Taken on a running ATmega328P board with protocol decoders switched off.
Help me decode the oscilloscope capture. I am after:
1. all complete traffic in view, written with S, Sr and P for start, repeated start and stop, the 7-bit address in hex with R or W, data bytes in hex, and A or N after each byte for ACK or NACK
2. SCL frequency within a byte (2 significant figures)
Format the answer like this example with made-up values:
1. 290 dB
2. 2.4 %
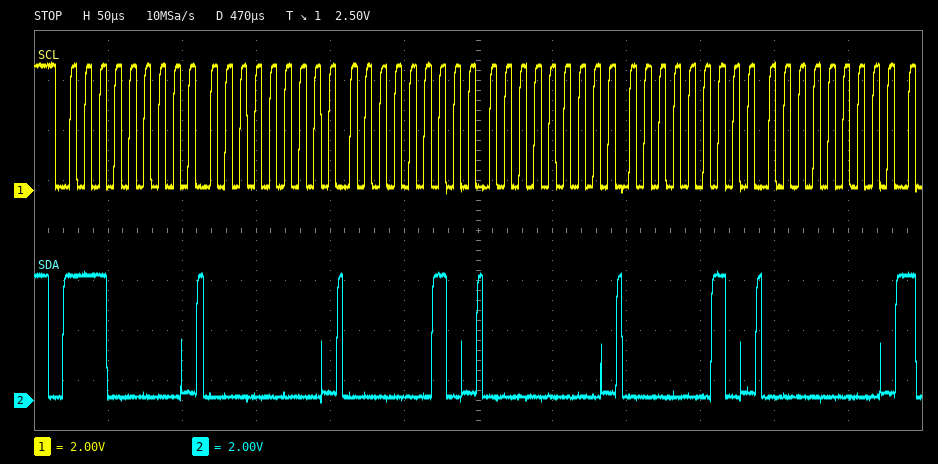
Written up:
1. S 70W A 00 A 02 A 00 A 02 A 00 A
2. 100 kHz
